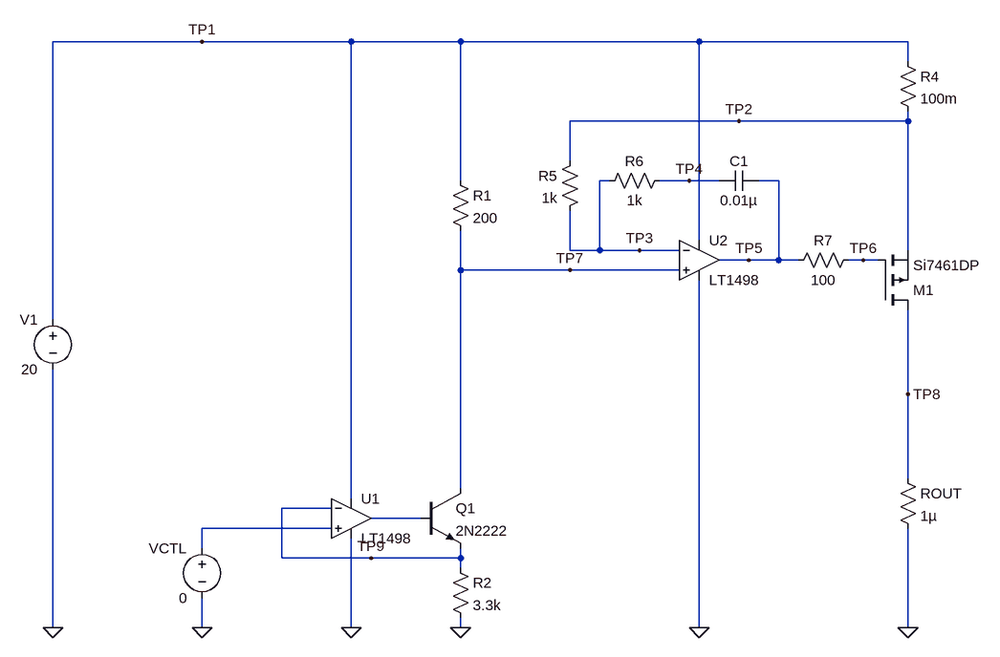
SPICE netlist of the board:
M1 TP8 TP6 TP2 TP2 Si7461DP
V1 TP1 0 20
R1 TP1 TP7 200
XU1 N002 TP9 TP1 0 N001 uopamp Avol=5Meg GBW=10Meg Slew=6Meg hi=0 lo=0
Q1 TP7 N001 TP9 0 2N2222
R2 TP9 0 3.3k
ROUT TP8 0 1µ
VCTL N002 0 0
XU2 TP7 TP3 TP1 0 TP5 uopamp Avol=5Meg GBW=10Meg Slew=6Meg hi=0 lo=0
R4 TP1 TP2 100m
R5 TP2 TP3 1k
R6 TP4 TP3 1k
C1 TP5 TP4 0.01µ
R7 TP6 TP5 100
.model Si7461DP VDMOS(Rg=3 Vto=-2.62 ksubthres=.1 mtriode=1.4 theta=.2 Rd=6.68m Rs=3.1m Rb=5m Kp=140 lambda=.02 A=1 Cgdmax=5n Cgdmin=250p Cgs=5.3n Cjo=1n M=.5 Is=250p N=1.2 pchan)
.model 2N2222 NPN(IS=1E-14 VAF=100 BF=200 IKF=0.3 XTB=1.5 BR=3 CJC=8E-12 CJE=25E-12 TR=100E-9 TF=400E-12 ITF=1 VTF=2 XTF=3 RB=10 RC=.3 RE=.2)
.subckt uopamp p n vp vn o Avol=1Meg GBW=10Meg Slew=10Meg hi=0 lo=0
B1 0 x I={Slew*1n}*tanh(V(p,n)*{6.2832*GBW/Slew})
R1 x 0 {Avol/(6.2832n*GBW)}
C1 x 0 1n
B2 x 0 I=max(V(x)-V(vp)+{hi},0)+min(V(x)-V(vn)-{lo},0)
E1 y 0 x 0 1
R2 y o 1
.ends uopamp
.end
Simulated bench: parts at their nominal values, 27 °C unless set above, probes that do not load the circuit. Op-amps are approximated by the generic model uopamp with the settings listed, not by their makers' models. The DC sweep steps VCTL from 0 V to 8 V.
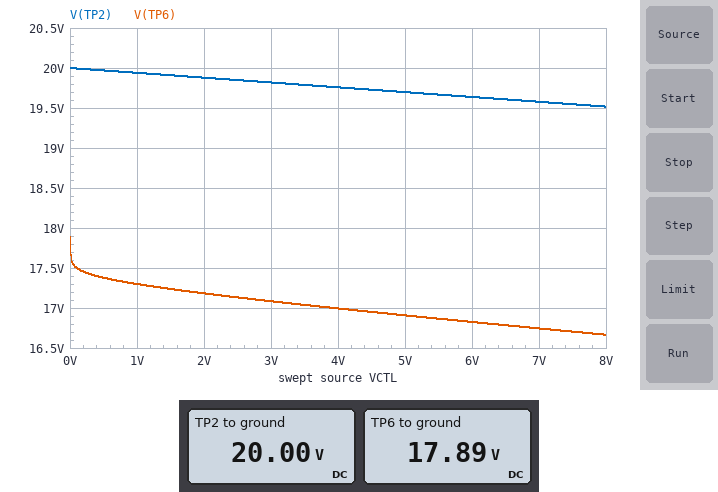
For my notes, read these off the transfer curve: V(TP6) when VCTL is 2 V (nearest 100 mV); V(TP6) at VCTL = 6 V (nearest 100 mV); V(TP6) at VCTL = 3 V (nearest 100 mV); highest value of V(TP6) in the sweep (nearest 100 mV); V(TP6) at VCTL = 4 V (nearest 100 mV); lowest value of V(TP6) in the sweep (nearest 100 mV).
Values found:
17.2 V
16.8 V
17.1 V
17.9 V
17.0 V
16.7 V
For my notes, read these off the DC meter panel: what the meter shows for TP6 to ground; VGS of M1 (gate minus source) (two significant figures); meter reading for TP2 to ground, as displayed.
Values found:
17.89 V
-2.1 V
20.00 V
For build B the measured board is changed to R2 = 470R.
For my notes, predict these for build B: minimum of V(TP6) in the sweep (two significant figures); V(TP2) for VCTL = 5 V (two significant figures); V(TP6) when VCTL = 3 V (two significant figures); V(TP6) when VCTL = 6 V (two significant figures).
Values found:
13 V
18 V
16 V
14 V
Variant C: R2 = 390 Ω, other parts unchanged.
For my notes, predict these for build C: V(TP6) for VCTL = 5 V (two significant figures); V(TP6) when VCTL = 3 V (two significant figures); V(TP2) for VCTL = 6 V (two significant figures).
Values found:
14 V
15 V
17 V
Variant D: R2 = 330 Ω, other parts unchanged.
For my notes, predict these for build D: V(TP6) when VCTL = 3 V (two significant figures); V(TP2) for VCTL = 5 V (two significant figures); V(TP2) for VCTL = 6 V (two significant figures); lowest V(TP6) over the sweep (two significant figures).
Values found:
15 V
17 V
16 V
12 V
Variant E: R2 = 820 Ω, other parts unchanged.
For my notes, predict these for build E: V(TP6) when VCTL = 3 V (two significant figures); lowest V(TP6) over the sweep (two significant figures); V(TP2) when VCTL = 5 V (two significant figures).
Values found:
16 V
15 V
19 V
